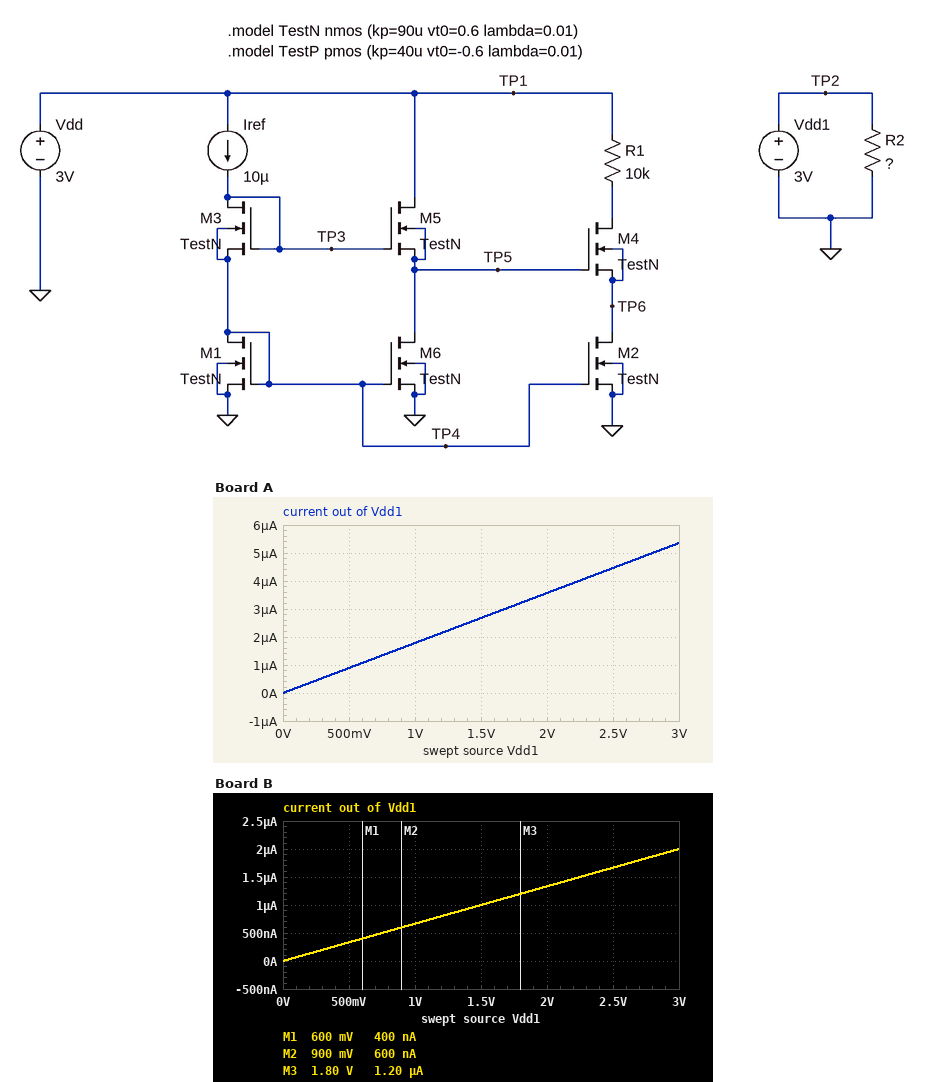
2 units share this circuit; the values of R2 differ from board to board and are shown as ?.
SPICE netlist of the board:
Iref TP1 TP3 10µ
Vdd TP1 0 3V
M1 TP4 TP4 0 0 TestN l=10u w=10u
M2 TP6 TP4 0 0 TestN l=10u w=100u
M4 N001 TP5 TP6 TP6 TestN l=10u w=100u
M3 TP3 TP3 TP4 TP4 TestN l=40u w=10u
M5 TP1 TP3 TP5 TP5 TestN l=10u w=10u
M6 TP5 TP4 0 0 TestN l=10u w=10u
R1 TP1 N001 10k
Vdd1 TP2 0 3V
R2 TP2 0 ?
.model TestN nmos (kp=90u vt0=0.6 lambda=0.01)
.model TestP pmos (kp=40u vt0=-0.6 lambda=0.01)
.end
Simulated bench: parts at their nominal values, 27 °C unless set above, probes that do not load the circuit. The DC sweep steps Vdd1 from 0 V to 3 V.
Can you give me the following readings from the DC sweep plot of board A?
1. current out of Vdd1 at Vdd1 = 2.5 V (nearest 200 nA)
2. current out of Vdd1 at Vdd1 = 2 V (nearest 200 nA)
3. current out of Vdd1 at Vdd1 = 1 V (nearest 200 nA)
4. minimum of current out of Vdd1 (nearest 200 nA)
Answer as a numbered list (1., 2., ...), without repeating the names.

1. 4.4 µA
2. 3.6 µA
3. 1.8 µA
4. 0 A
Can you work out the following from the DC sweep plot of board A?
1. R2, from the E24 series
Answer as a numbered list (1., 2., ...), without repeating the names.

1. 560 kΩ
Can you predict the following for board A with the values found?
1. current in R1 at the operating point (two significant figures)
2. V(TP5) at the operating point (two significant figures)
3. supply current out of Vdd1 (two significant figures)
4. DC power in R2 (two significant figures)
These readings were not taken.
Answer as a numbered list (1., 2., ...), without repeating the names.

1. 99 µA
2. 1.5 V
3. 5.4 µA
4. 16 µW
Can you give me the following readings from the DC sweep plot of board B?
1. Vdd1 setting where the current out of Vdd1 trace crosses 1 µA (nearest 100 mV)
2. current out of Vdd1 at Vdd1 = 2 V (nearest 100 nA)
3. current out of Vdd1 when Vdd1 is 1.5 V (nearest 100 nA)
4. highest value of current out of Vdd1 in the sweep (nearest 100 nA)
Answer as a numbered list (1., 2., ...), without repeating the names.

1. 1.5 V
2. 1.3 µA
3. 1.0 µA
4. 2.0 µA
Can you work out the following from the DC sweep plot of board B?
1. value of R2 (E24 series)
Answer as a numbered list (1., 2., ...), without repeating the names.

1. 1.5 MΩ
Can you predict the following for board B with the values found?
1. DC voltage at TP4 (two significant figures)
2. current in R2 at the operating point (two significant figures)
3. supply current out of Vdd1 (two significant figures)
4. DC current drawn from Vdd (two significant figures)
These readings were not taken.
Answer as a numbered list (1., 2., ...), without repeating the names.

1. 1.1 V
2. 2.0 µA
3. 2.0 µA
4. 120 µA
